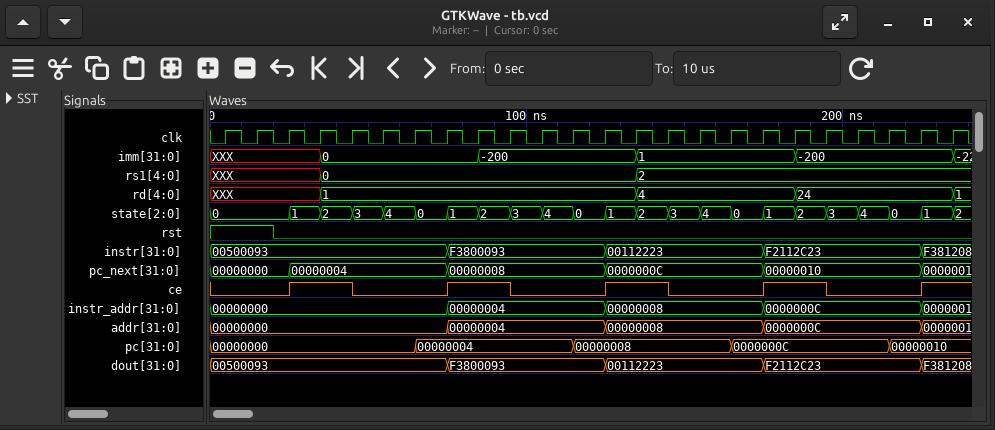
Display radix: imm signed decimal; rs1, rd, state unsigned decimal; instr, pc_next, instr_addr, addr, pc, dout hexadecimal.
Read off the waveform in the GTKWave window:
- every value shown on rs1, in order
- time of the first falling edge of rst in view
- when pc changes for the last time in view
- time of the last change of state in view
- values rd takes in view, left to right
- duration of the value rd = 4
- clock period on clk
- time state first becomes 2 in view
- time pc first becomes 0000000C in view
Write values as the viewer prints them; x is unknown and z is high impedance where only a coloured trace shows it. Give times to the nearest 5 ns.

XXX, 0, 2
20 ns
215 ns
235 ns
XXX, 1, 4, 24, 1
50 ns
10 ns
35 ns
165 ns
